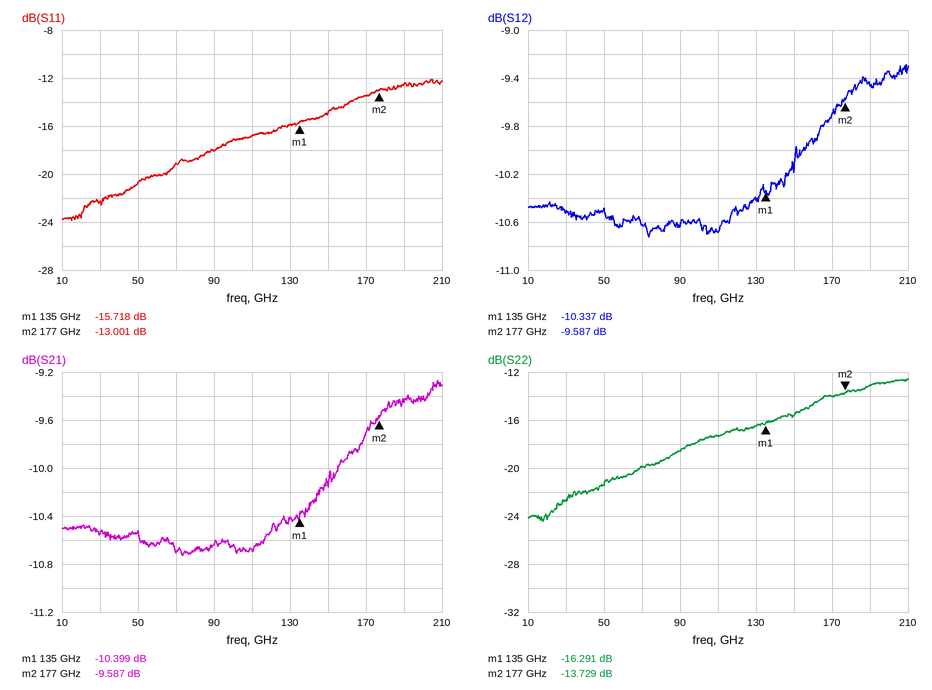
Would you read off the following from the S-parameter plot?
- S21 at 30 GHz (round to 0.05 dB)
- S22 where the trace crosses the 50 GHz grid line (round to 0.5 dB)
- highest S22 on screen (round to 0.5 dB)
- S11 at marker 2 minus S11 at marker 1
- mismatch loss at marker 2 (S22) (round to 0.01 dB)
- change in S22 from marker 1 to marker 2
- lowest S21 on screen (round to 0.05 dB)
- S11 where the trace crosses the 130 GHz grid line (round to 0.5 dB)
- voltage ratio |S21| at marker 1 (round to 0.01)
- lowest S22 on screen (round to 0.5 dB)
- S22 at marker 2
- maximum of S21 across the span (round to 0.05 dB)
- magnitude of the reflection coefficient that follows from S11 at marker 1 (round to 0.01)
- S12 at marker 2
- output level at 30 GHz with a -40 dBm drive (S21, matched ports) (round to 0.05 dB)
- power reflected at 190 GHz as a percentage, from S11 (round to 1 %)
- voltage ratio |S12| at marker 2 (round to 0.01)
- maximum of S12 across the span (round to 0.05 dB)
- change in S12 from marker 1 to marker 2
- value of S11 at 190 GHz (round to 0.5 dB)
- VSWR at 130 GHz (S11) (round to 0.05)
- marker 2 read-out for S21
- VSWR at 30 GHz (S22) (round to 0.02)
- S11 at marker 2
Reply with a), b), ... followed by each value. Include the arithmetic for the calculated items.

a) -10.55 dB
b) -21.5 dB
c) -12.5 dB
d) -13.001 − (-15.718) = 2.717 dB
e) −10 log10(1 − 10^(-13.729/10)) ≈ 0.19 dB
f) -13.729 − (-16.291) = 2.562 dB
g) -10.75 dB
h) -16.0 dB
i) 10^(-10.399/20) ≈ 0.30
j) -24.5 dB
k) -13.729 dB
l) -9.25 dB
m) 10^(-15.718/20) ≈ 0.16
n) -9.587 dB
o) -40 dBm + (-10.55 dB) = -50.55 dBm
p) 10^(-12.5/10) ≈ 6 %
q) 10^(-9.587/20) ≈ 0.33
r) -9.30 dB
s) -9.587 − (-10.337) = 0.750 dB
t) -12.5 dB
u) |Γ| = 10^(-16/20) = 0.1585; VSWR = (1 + 0.1585)/(1 − 0.1585) ≈ 1.38, so 1.40 to the nearest 0.05
v) -9.587 dB
w) |Γ| = 10^(-22.5/20) = 0.0750; VSWR = (1 + 0.0750)/(1 − 0.0750) ≈ 1.16
x) -13.001 dB
